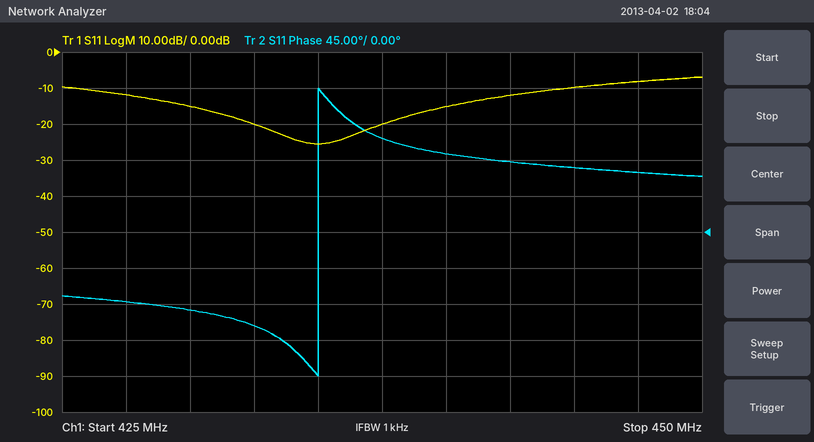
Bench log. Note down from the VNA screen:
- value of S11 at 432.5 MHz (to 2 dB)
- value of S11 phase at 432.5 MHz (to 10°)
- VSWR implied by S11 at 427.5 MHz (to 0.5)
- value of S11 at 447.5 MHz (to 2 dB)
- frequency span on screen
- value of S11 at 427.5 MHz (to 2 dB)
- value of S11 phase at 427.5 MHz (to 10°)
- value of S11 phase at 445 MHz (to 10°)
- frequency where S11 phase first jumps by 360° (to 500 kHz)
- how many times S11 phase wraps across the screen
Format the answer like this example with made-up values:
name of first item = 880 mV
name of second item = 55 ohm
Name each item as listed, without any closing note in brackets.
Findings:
value of S11 at 432.5 MHz = -20 dB
value of S11 phase at 432.5 MHz = -120°
VSWR implied by S11 at 427.5 MHz = 1.5
value of S11 at 447.5 MHz = -8 dB
frequency span on screen = 25 MHz
value of S11 at 427.5 MHz = -12 dB
value of S11 phase at 427.5 MHz = -90°
value of S11 phase at 445 MHz = 80°
frequency where S11 phase first jumps by 360° = 435.0 MHz
how many times S11 phase wraps across the screen = 1
